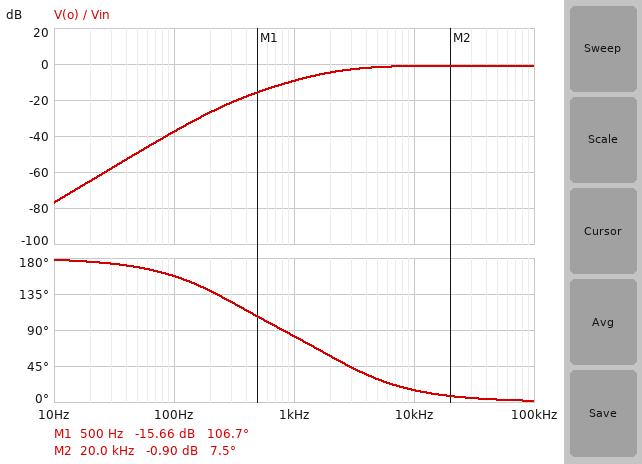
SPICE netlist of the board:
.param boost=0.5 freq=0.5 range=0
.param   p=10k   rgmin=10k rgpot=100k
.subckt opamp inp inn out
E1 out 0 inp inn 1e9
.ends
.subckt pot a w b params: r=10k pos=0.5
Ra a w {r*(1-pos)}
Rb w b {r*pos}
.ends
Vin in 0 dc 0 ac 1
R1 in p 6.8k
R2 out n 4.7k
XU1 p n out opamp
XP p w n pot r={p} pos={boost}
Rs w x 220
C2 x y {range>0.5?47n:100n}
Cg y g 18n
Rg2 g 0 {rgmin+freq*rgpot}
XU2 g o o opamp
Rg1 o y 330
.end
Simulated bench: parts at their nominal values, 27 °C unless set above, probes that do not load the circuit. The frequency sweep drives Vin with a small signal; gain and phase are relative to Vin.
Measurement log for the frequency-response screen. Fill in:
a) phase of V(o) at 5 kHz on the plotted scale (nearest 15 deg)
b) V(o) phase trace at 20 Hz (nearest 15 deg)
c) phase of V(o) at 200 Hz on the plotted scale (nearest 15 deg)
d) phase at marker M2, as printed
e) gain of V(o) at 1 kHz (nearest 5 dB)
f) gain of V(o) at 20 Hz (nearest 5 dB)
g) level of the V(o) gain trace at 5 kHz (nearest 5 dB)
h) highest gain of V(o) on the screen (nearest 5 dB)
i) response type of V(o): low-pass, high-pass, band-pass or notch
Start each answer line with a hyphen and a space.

- 30 deg
- 180 deg
- 135 deg
- 7.5 deg
- -10 dB
- -65 dB
- 0 dB
- 0 dB
- high-pass
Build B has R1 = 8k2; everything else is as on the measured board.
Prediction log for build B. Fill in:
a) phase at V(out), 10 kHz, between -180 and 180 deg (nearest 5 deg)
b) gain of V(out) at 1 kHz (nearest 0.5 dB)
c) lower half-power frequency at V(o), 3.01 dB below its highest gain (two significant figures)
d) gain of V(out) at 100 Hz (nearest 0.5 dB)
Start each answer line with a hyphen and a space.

- 5 deg
- -2.5 dB
- 2.7 kHz
- -0.5 dB
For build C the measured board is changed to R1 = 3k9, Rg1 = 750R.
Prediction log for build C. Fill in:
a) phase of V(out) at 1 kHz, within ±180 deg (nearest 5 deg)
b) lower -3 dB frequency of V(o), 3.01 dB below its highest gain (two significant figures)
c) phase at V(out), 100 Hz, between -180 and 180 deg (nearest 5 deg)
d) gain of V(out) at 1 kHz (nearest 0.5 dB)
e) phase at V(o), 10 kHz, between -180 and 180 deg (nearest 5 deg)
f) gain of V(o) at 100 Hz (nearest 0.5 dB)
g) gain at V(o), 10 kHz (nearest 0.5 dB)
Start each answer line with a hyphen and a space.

- 0 deg
- 770 Hz
- 0 deg
- 0.5 dB
- 5 deg
- -30.0 dB
- -0.5 dB
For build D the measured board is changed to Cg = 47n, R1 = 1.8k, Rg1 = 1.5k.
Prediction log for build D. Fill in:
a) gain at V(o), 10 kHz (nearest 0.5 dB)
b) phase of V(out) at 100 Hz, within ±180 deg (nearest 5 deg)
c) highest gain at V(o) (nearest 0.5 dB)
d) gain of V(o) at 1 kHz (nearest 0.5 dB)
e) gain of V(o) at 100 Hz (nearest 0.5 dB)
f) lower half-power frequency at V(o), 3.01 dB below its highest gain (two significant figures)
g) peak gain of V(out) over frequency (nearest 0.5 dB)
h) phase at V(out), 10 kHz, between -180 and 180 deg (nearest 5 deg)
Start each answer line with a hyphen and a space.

- -0.5 dB
- 5 deg
- 1.5 dB
- 0 dB
- -14.5 dB
- 200 Hz
- 2.0 dB
- 0 deg
